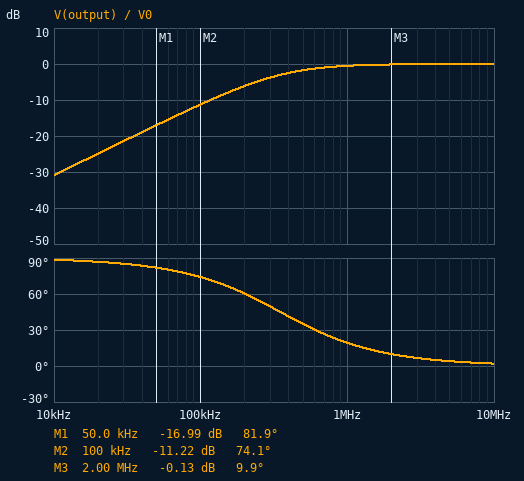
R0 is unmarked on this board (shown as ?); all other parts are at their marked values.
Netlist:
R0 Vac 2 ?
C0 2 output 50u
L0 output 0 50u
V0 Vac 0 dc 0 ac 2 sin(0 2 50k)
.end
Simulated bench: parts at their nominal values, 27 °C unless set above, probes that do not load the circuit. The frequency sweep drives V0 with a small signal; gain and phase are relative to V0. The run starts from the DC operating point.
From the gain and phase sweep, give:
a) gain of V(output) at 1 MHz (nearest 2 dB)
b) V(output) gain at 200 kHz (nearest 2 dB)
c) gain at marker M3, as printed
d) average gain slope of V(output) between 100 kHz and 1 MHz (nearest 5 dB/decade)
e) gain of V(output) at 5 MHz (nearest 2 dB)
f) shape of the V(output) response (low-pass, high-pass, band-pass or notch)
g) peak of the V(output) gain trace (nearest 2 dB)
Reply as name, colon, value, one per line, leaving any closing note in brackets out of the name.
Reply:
gain of V(output) at 1 MHz: 0 dB
V(output) gain at 200 kHz: -6 dB
gain at marker M3, as printed: -0.13 dB
average gain slope of V(output) between 100 kHz and 1 MHz: 10 dB/decade
gain of V(output) at 5 MHz: 0 dB
shape of the V(output) response: high-pass
peak of the V(output) gain trace: 0 dB
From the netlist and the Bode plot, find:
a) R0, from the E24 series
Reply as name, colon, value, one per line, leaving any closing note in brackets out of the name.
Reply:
R0, from the E24 series: 110 Ω
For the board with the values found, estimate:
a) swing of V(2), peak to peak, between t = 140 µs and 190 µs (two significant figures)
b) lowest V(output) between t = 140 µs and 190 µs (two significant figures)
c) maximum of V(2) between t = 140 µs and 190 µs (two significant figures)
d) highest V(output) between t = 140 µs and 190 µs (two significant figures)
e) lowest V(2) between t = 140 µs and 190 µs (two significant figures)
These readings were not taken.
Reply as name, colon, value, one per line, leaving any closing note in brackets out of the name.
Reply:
swing of V(2), peak to peak, between t = 140 µs and 190 µs: 560 mV
lowest V(output) between t = 140 µs and 190 µs: -280 mV
maximum of V(2) between t = 140 µs and 190 µs: 280 mV
highest V(output) between t = 140 µs and 190 µs: 280 mV
lowest V(2) between t = 140 µs and 190 µs: -280 mV
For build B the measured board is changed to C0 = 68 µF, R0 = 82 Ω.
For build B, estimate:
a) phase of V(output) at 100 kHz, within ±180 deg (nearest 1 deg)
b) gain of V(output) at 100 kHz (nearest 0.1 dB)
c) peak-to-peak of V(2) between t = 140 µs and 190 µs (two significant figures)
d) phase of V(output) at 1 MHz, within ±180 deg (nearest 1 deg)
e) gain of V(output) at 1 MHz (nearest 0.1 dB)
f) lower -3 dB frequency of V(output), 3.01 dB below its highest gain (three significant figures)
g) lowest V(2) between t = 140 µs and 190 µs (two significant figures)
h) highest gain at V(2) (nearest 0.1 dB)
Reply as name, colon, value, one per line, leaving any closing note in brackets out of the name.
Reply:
phase of V(output) at 100 kHz, within ±180 deg: 69 deg
gain of V(output) at 100 kHz: -8.9 dB
peak-to-peak of V(2) between t = 140 µs and 190 µs: 750 mV
phase of V(output) at 1 MHz, within ±180 deg: 15 deg
gain of V(output) at 1 MHz: -0.3 dB
lower -3 dB frequency of V(output), 3.01 dB below its highest gain: 261 kHz
lowest V(2) between t = 140 µs and 190 µs: -370 mV
highest gain at V(2): 0 dB
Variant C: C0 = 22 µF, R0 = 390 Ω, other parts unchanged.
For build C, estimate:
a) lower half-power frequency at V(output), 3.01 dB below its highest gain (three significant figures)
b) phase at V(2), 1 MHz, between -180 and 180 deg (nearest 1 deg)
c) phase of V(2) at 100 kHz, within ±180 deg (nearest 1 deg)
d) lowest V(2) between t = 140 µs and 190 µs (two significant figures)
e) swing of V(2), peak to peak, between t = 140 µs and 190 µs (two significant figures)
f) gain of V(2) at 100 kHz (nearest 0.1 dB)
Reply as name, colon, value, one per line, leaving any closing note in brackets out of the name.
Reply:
lower half-power frequency at V(output), 3.01 dB below its highest gain: 1.24 MHz
phase at V(2), 1 MHz, between -180 and 180 deg: 51 deg
phase of V(2) at 100 kHz, within ±180 deg: 85 deg
lowest V(2) between t = 140 µs and 190 µs: -79 mV
swing of V(2), peak to peak, between t = 140 µs and 190 µs: 160 mV
gain of V(2) at 100 kHz: -21.9 dB
